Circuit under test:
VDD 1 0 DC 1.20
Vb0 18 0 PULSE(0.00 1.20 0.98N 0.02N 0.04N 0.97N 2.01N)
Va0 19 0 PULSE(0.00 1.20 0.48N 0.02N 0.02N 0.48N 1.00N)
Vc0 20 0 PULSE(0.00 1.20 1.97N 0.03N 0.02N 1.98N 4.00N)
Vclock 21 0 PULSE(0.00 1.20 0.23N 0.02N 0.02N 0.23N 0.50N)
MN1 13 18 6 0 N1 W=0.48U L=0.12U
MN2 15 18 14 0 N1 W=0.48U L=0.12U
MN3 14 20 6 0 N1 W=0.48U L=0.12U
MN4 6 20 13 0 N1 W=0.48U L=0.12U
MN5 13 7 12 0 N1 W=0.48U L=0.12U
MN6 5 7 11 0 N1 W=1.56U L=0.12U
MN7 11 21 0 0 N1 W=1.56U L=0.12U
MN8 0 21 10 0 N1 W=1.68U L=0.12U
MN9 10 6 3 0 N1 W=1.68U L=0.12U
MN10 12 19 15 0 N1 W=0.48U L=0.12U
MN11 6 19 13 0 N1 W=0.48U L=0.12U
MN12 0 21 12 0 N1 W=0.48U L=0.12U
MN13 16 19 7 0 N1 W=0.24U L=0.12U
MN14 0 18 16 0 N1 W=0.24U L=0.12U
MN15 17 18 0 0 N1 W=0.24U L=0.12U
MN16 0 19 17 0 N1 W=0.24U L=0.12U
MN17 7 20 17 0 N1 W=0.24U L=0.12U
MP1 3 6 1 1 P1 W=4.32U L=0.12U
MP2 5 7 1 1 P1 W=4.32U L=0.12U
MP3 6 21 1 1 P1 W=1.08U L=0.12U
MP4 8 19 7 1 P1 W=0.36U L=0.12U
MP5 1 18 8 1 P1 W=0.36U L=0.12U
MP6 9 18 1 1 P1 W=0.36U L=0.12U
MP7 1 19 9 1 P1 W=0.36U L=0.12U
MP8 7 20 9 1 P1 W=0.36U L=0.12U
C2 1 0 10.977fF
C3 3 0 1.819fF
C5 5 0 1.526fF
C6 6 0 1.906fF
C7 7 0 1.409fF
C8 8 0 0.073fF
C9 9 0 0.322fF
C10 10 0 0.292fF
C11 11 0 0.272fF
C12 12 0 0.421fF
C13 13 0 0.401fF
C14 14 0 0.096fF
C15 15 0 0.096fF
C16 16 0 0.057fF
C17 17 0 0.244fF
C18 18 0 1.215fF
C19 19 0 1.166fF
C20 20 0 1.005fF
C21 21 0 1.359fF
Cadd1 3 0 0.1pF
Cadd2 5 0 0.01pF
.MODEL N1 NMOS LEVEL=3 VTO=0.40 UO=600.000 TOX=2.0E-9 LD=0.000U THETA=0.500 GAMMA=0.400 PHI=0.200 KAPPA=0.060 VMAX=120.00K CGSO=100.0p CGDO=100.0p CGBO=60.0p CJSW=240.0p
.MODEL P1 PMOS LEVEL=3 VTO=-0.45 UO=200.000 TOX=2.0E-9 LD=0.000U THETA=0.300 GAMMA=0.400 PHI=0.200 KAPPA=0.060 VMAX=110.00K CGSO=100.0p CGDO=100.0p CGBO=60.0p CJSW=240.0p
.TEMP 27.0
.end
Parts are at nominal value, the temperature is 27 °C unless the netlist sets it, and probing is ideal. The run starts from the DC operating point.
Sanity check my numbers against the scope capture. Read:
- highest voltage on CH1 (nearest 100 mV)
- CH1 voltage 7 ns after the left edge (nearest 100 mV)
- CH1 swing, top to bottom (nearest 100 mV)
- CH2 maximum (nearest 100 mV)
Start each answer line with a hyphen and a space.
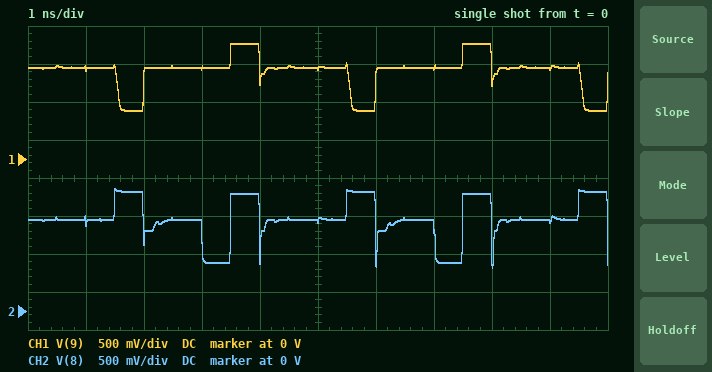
- 1.5 V
- 1.2 V
- 900 mV
- 1.6 V
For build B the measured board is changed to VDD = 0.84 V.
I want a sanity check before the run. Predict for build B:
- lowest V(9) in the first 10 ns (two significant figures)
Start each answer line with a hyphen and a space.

- 550 mV
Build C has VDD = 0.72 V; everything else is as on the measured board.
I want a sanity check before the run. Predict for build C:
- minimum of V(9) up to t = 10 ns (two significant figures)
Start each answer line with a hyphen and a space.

- 530 mV
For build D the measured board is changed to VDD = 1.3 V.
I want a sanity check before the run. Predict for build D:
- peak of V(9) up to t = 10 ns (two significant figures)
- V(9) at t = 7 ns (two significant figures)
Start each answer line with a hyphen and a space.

- 1.6 V
- 1.3 V
